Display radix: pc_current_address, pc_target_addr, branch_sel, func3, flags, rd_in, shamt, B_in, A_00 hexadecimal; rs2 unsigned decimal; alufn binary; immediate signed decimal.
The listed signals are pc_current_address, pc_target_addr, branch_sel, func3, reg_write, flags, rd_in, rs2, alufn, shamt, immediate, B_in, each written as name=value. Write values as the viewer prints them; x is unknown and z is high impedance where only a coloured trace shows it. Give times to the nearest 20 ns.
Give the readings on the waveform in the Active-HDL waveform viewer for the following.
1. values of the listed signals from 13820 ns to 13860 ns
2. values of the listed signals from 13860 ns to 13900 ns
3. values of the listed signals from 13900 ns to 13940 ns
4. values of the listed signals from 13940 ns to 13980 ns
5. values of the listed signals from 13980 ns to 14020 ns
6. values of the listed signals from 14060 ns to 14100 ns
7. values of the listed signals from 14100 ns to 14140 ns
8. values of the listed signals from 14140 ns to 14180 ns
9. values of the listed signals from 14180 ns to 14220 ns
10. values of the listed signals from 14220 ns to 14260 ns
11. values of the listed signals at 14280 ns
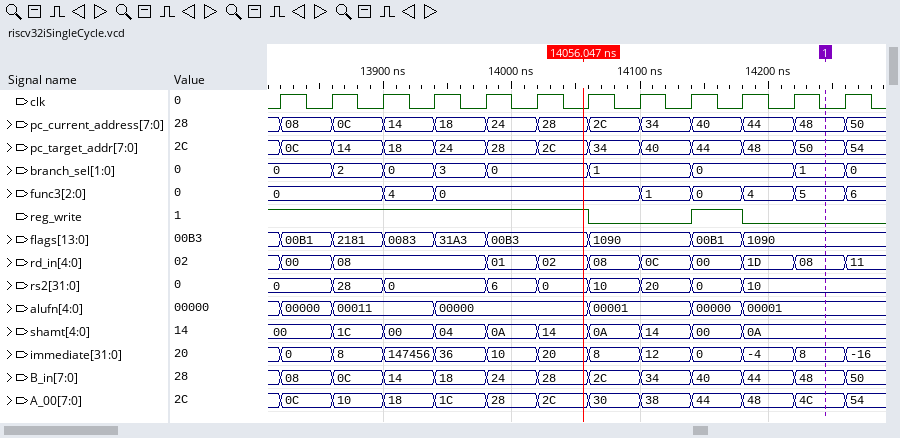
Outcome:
pc_current_address=08, pc_target_addr=0C, branch_sel=0, func3=0, reg_write=1, flags=00B1, rd_in=00, rs2=0, alufn=00000, shamt=00, immediate=0, B_in=08
pc_current_address=0C, pc_target_addr=14, branch_sel=2, func3=0, reg_write=1, flags=2181, rd_in=08, rs2=28, alufn=00011, shamt=1C, immediate=8, B_in=0C
pc_current_address=14, pc_target_addr=18, branch_sel=0, func3=4, reg_write=1, flags=0083, rd_in=08, rs2=0, alufn=00011, shamt=00, immediate=147456, B_in=14
pc_current_address=18, pc_target_addr=24, branch_sel=3, func3=0, reg_write=1, flags=31A3, rd_in=08, rs2=0, alufn=00000, shamt=04, immediate=36, B_in=18
pc_current_address=24, pc_target_addr=28, branch_sel=0, func3=0, reg_write=1, flags=00B3, rd_in=01, rs2=6, alufn=00000, shamt=0A, immediate=10, B_in=24
pc_current_address=2C, pc_target_addr=34, branch_sel=1, func3=0, reg_write=0, flags=1090, rd_in=08, rs2=10, alufn=00001, shamt=0A, immediate=8, B_in=2C
pc_current_address=34, pc_target_addr=40, branch_sel=1, func3=1, reg_write=0, flags=1090, rd_in=0C, rs2=20, alufn=00001, shamt=14, immediate=12, B_in=34
pc_current_address=40, pc_target_addr=44, branch_sel=0, func3=0, reg_write=1, flags=00B1, rd_in=00, rs2=0, alufn=00000, shamt=00, immediate=0, B_in=40
pc_current_address=44, pc_target_addr=48, branch_sel=0, func3=4, reg_write=0, flags=1090, rd_in=1D, rs2=10, alufn=00001, shamt=0A, immediate=-4, B_in=44
pc_current_address=48, pc_target_addr=50, branch_sel=1, func3=5, reg_write=0, flags=1090, rd_in=08, rs2=10, alufn=00001, shamt=0A, immediate=8, B_in=48
pc_current_address=50, pc_target_addr=54, branch_sel=0, func3=6, reg_write=0, flags=1090, rd_in=11, rs2=10, alufn=00001, shamt=0A, immediate=-16, B_in=50
